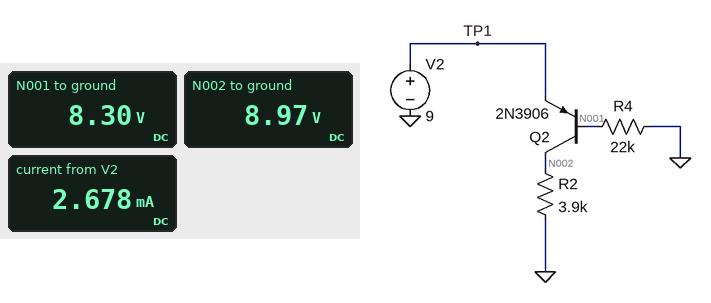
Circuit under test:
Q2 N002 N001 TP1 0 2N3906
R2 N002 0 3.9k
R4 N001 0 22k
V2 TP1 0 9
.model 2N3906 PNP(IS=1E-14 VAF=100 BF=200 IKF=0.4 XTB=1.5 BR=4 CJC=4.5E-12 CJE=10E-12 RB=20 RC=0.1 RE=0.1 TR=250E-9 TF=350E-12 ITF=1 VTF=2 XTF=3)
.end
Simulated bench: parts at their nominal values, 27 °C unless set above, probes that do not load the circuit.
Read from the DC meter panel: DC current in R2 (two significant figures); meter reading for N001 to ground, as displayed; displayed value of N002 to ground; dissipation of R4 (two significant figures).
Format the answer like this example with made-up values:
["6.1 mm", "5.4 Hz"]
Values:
["2.3 mA", "8.30 V", "8.97 V", "3.1 mW"]
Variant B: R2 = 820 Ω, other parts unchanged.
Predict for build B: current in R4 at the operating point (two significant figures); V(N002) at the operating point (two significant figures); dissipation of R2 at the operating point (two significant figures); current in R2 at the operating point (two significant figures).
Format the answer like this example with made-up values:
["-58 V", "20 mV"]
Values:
["380 µA", "8.9 V", "97 mW", "11 mA"]
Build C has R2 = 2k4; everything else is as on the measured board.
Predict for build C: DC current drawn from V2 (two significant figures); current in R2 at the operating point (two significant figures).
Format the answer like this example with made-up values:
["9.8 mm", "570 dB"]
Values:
["4.1 mA", "3.7 mA"]
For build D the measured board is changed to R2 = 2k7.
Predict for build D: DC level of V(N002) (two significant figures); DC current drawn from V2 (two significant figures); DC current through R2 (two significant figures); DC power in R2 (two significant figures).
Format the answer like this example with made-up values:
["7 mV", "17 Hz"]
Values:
["9.0 V", "3.7 mA", "3.3 mA", "30 mW"]
